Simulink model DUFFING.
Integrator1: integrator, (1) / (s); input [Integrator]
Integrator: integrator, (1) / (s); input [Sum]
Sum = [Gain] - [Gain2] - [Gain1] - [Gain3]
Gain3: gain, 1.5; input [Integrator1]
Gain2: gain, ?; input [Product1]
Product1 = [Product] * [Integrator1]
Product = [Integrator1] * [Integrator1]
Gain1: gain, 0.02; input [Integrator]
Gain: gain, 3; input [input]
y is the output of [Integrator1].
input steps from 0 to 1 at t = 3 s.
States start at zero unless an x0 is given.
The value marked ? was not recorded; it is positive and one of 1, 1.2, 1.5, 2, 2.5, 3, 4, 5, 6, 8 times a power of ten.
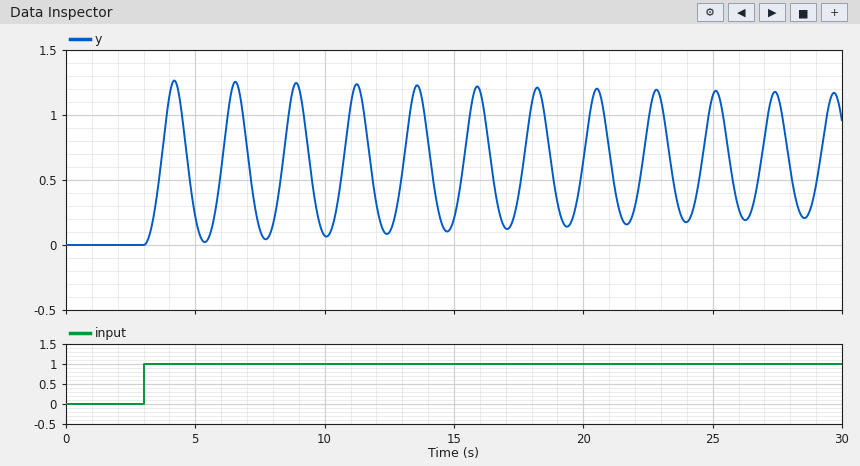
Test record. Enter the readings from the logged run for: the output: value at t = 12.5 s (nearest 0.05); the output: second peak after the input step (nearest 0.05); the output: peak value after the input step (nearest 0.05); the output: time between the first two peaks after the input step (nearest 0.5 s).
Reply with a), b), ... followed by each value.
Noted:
a) 0.10
b) 1.25
c) 1.25
d) 2.5 s
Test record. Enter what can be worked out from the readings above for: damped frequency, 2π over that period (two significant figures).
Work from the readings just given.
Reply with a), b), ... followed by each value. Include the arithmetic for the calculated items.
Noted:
a) 2π / 2.5 = 2.5 rad/s
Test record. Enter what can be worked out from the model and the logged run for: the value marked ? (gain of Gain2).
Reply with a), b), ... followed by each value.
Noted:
a) 4
